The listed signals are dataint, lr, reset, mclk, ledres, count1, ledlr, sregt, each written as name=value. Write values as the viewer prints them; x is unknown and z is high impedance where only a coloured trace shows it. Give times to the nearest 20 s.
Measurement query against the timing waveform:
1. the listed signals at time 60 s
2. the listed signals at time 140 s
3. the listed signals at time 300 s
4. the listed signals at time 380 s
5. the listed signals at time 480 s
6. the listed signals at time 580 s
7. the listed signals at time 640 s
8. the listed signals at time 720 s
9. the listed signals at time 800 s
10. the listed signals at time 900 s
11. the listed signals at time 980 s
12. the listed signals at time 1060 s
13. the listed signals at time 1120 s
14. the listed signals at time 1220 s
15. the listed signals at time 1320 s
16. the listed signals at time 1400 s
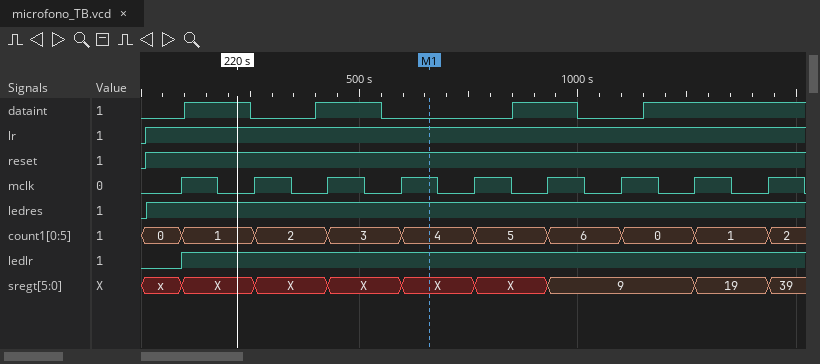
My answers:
dataint=0, lr=1, reset=1, mclk=0, ledres=1, count1=0, ledlr=0, sregt=x
dataint=1, lr=1, reset=1, mclk=1, ledres=1, count1=1, ledlr=1, sregt=X
dataint=0, lr=1, reset=1, mclk=1, ledres=1, count1=2, ledlr=1, sregt=X
dataint=0, lr=1, reset=1, mclk=0, ledres=1, count1=2, ledlr=1, sregt=X
dataint=1, lr=1, reset=1, mclk=1, ledres=1, count1=3, ledlr=1, sregt=X
dataint=0, lr=1, reset=1, mclk=0, ledres=1, count1=3, ledlr=1, sregt=X
dataint=0, lr=1, reset=1, mclk=1, ledres=1, count1=4, ledlr=1, sregt=X
dataint=0, lr=1, reset=1, mclk=0, ledres=1, count1=4, ledlr=1, sregt=X
dataint=0, lr=1, reset=1, mclk=1, ledres=1, count1=5, ledlr=1, sregt=X
dataint=1, lr=1, reset=1, mclk=0, ledres=1, count1=5, ledlr=1, sregt=X
dataint=1, lr=1, reset=1, mclk=1, ledres=1, count1=6, ledlr=1, sregt=9
dataint=0, lr=1, reset=1, mclk=0, ledres=1, count1=6, ledlr=1, sregt=9
dataint=0, lr=1, reset=1, mclk=1, ledres=1, count1=0, ledlr=1, sregt=9
dataint=1, lr=1, reset=1, mclk=0, ledres=1, count1=0, ledlr=1, sregt=9
dataint=1, lr=1, reset=1, mclk=1, ledres=1, count1=1, ledlr=1, sregt=19
dataint=1, lr=1, reset=1, mclk=0, ledres=1, count1=1, ledlr=1, sregt=19
